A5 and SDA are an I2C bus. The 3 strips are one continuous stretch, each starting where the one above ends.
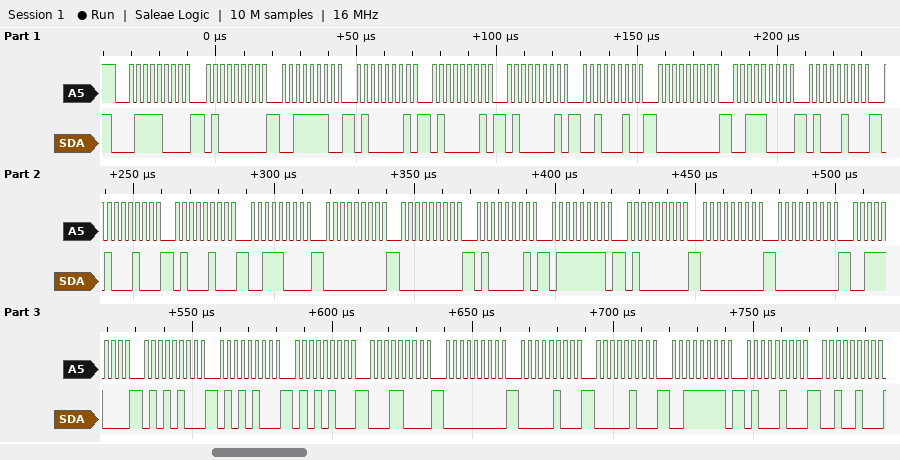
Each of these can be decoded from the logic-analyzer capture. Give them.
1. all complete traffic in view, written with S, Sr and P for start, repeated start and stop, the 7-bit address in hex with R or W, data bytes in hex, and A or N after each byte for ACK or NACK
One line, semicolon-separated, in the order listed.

S 3CW A 40 A 3E A 41 A 41 A 41 A 22 A 00 A 38 A 44 A 44 A 44 A 38 A 00 A 00 A 41 A 7F A 40 A 00 A 00 A 38 A 54 A 54 A 54 A 18 A 00 A 04 A 04 A 3F A 44 A 24 A
